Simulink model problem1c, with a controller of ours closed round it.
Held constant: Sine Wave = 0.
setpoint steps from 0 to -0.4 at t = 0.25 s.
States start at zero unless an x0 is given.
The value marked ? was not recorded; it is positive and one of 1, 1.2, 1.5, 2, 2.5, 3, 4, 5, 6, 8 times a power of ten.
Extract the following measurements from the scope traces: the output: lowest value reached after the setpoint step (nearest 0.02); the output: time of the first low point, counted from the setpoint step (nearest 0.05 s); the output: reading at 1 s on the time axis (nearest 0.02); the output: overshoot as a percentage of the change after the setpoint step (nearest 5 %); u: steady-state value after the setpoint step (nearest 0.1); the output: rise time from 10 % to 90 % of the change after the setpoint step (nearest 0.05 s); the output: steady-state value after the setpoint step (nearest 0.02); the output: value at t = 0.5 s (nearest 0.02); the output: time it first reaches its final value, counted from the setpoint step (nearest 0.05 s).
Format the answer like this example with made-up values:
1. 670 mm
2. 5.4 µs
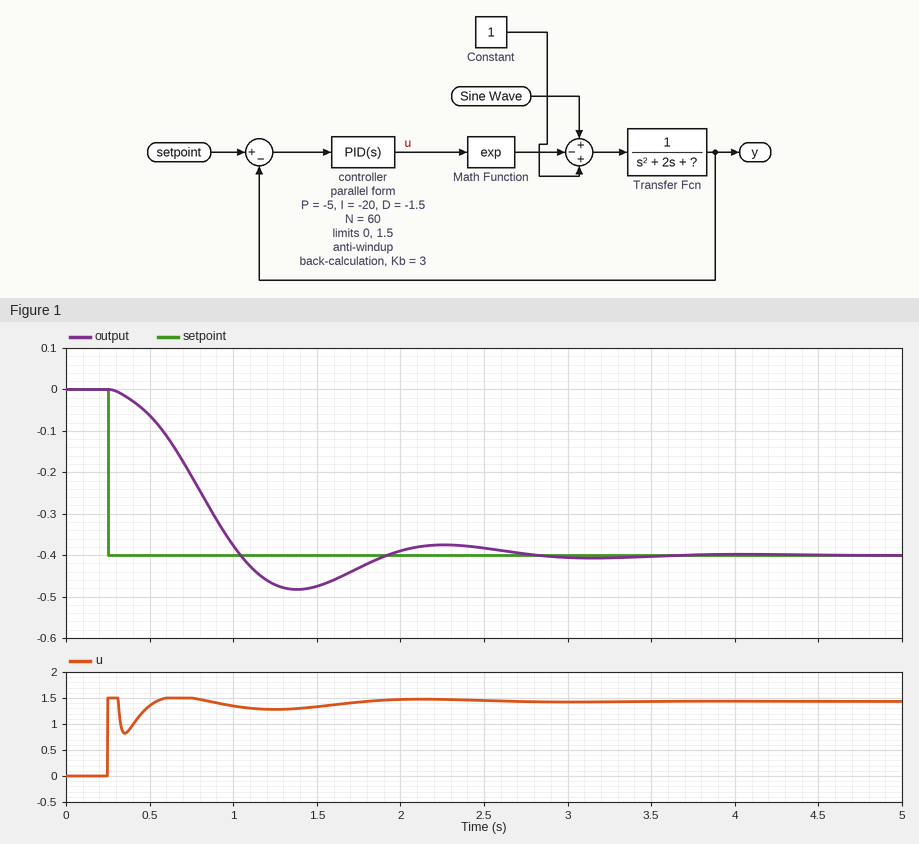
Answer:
1. -0.48
2. 1.15 s
3. -0.38
4. 20 %
5. 1.4
6. 0.55 s
7. -0.40
8. -0.06
9. 0.80 s
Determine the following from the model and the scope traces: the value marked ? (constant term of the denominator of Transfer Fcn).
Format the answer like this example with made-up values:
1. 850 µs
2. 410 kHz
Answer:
1. 8
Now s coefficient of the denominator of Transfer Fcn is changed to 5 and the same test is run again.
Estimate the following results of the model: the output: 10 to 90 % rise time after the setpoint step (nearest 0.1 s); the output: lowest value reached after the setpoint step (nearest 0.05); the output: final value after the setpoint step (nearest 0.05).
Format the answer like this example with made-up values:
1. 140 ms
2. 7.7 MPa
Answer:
1. 0.9 s
2. -0.45
3. -0.40
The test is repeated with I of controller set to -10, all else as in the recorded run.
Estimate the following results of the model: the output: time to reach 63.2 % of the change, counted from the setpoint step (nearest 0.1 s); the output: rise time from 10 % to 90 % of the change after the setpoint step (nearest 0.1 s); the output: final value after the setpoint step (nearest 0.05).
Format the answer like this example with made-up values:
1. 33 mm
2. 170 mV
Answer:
1. 0.9 s
2. 1.1 s
3. -0.40
